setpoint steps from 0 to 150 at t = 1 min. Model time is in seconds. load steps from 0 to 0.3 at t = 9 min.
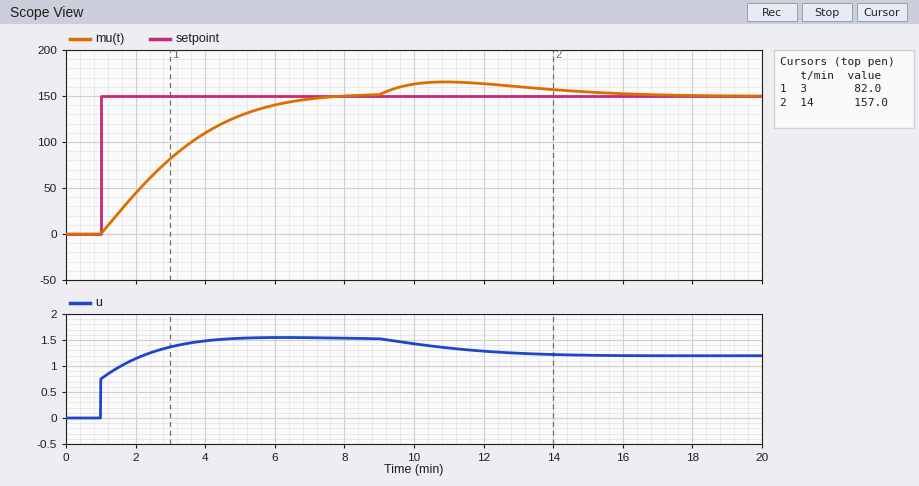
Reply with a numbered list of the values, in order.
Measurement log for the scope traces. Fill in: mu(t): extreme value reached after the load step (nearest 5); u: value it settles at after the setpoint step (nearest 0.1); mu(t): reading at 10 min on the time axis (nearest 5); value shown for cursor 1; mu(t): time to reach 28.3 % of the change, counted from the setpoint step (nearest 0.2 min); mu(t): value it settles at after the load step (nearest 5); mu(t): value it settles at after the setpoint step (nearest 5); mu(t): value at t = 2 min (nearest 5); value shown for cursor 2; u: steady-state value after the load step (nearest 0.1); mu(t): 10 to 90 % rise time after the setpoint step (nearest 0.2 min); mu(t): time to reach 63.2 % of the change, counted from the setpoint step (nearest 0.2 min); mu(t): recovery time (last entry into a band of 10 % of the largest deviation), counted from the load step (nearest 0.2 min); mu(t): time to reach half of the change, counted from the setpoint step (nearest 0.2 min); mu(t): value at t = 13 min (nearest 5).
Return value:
1. 165
2. 1.5
3. 165
4. 82.0
5. 1.0 min
6. 150
7. 150
8. 45
9. 157.0
10. 1.2
11. 4.2 min
12. 2.4 min
13. 7.8 min
14. 1.8 min
15. 160
